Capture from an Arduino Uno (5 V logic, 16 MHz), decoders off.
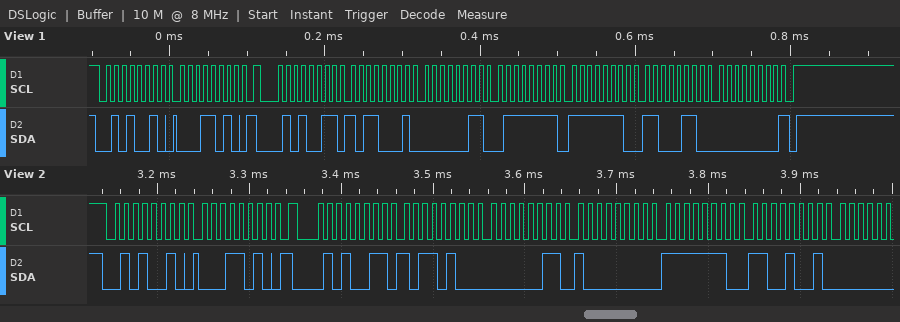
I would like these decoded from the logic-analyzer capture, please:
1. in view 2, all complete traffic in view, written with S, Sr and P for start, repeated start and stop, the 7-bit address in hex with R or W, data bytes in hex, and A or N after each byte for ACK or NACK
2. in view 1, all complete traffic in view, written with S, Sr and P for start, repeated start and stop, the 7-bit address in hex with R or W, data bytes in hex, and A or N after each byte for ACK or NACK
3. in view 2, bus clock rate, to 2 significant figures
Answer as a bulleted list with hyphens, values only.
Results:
- S 29W A 1A A Sr 29R A B4 A 03 A 80 A FE A C9 A
- S 29W A 1A A Sr 29R A B1 A 03 A 7F A FE A C6 A 00 N P
- 100 kHz
